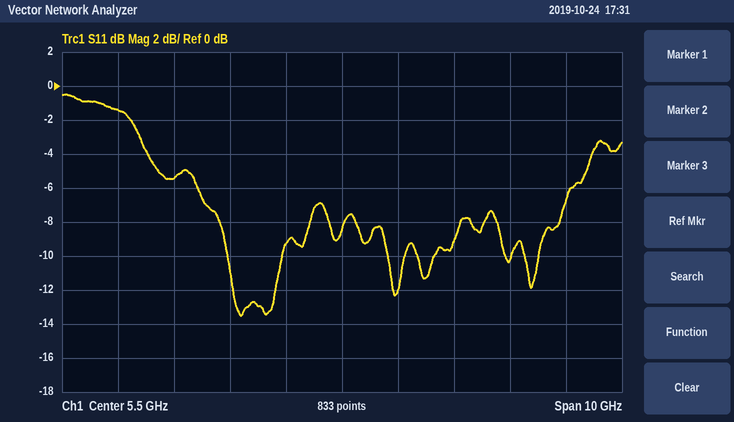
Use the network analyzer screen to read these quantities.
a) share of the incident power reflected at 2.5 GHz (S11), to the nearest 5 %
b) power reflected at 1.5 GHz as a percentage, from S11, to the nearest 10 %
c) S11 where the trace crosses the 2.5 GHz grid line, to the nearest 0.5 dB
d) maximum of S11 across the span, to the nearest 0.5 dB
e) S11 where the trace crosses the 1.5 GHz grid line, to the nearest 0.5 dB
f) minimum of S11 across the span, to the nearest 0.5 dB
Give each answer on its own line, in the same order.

30 %
70 %
-5.5 dB
-0.5 dB
-1.5 dB
-13.5 dB
